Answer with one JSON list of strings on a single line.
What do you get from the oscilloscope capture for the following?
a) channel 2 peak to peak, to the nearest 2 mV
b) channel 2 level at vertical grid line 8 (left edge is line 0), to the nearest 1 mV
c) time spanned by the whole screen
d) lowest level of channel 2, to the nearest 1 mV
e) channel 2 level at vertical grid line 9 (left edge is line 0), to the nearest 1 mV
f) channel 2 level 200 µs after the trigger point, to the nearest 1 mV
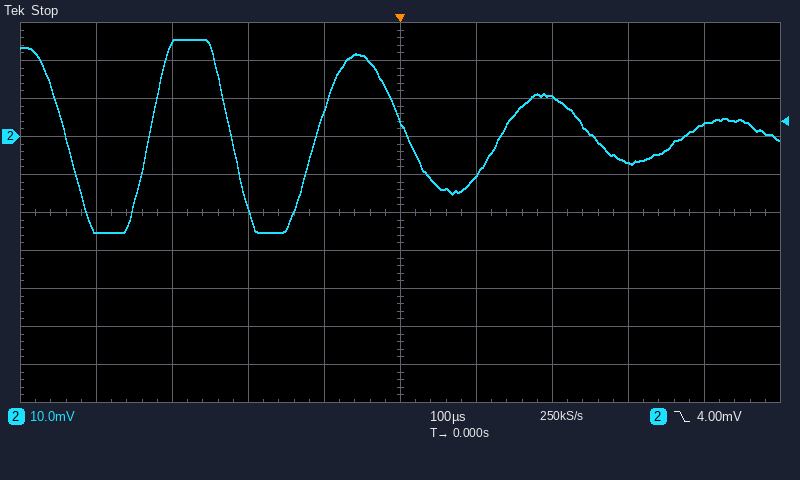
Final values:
["50 mV", "-7 mV", "1 ms", "-25 mV", "3 mV", "10 mV"]
